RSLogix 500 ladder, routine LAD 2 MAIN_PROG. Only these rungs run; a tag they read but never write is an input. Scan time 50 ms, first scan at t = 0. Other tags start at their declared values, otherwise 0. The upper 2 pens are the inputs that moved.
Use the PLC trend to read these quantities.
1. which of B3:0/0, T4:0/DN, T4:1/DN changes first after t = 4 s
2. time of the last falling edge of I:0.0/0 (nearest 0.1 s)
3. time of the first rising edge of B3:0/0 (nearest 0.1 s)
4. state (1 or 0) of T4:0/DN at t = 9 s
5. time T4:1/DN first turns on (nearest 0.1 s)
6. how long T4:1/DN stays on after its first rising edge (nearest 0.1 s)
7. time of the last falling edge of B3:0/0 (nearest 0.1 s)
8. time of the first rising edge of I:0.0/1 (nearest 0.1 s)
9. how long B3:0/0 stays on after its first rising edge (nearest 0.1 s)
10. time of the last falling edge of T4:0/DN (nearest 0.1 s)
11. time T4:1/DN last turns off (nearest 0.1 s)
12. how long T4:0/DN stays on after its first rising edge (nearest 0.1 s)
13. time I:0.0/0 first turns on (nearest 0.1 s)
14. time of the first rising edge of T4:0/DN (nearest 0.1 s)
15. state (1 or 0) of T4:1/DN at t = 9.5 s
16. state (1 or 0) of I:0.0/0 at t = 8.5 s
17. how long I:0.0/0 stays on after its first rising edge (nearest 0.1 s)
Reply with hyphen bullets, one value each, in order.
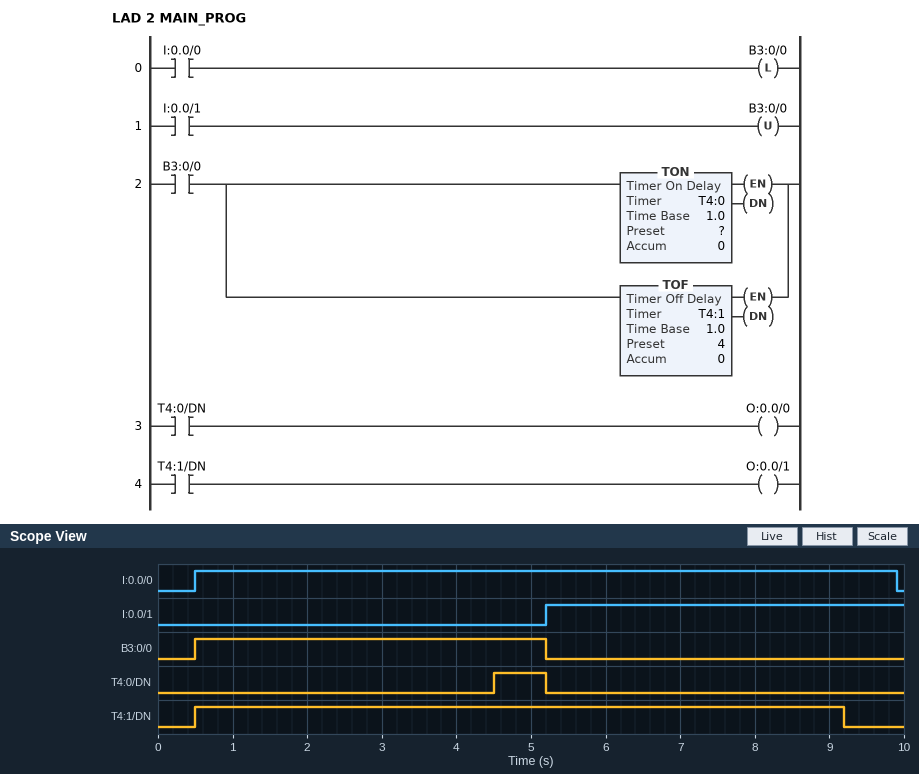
- T4:0/DN
- 9.9 s
- 0.5 s
- 0
- 0.5 s
- 8.7 s
- 5.2 s
- 5.2 s
- 4.7 s
- 5.2 s
- 9.2 s
- 0.7 s
- 0.5 s
- 4.5 s
- 0
- 1
- 9.4 s
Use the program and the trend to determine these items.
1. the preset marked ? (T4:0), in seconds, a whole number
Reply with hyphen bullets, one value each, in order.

- 4 s
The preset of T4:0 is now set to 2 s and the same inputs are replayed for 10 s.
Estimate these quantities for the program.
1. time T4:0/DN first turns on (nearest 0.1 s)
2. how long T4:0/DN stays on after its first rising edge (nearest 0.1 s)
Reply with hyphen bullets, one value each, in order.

- 2.5 s
- 2.7 s
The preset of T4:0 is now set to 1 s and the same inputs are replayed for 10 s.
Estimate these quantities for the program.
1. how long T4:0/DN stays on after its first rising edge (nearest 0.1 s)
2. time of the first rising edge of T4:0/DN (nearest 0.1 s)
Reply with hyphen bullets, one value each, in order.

- 3.7 s
- 1.5 s
